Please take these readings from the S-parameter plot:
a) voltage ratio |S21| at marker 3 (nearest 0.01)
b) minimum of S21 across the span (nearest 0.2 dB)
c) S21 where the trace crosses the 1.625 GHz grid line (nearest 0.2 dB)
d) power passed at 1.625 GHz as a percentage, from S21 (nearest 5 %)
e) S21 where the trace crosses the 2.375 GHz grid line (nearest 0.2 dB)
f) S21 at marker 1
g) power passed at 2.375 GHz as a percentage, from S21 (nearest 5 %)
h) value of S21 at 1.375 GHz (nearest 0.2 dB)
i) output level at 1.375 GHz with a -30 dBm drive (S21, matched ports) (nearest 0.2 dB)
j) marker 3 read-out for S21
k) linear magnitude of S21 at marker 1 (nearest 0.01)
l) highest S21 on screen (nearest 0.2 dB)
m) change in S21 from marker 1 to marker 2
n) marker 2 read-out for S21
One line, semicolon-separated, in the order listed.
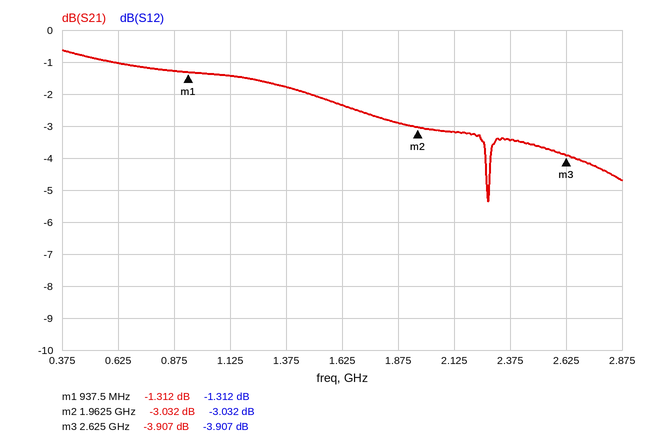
0.64; -5.4 dB; -2.4 dB; 60 %; -3.4 dB; -1.312 dB; 45 %; -1.8 dB; -31.8 dBm; -3.907 dB; 0.86; -0.6 dB; -1.720 dB; -3.032 dB
